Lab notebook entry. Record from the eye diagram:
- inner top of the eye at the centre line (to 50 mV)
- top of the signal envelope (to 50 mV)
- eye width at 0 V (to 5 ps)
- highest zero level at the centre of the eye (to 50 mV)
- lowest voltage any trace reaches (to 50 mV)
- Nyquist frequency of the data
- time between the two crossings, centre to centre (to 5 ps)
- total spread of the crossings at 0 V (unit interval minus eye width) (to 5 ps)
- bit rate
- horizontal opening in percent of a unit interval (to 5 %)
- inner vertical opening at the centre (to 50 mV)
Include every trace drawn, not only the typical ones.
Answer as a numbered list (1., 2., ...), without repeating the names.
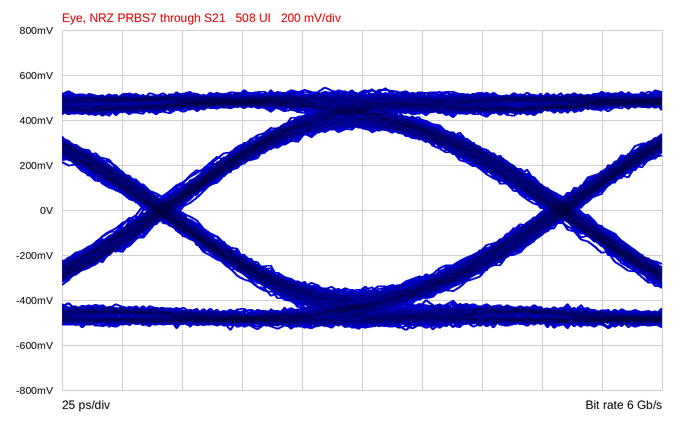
1. 350 mV
2. 550 mV
3. 150 ps
4. -350 mV
5. -550 mV
6. 3 GHz
7. 165 ps
8. 15 ps
9. 6 Gb/s
10. 90 %
11. 700 mV
